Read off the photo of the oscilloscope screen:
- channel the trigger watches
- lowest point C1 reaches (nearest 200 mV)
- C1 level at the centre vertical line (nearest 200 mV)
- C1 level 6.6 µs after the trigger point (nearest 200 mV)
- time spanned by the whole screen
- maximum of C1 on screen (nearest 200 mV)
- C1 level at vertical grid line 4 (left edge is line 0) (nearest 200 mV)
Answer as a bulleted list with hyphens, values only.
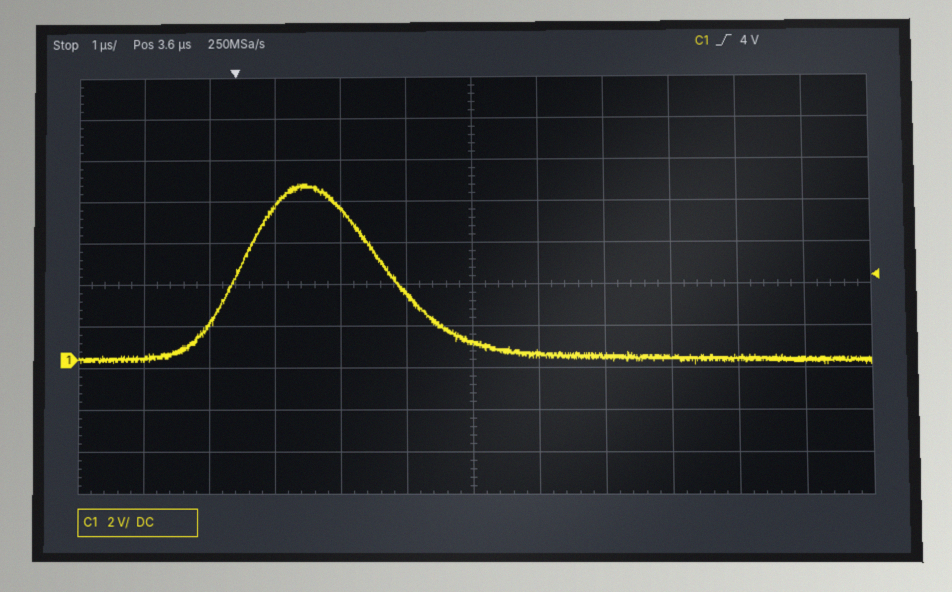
- C1
- -200 mV
- 800 mV
- 200 mV
- 12 µs
- 8.4 V
- 7.2 V
